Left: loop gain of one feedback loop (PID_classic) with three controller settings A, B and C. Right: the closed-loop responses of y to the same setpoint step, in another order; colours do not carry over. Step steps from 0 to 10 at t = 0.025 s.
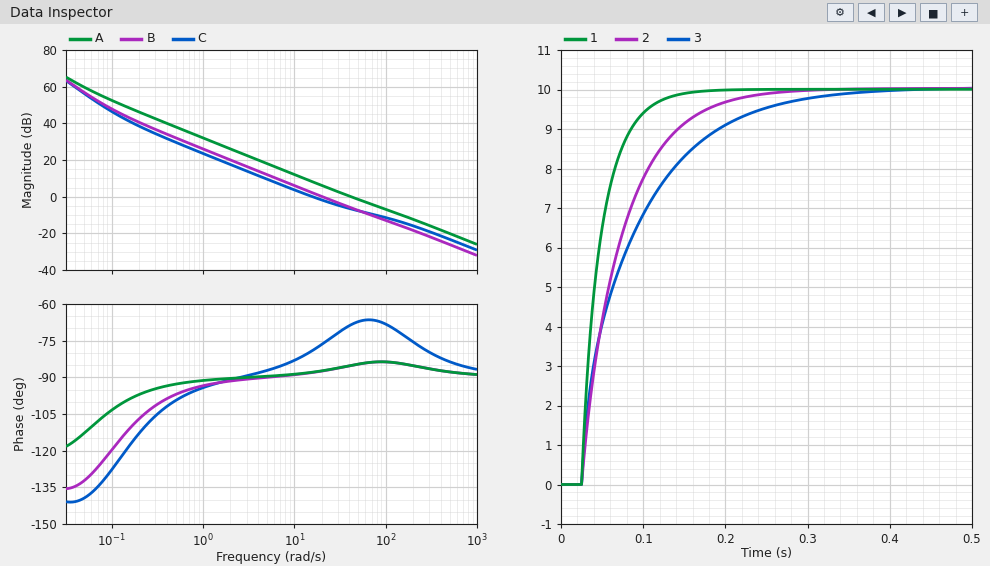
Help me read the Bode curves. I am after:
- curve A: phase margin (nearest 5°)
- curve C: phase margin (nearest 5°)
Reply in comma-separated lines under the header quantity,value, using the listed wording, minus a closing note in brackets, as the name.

quantity,value
curve A: phase margin,95°
curve C: phase margin,100°
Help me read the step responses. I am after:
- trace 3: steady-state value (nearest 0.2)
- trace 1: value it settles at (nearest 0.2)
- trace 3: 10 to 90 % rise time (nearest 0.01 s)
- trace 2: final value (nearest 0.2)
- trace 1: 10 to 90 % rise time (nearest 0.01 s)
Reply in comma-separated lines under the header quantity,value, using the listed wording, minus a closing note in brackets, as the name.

quantity,value
trace 3: steady-state value,10.0
trace 1: value it settles at,10.0
trace 3: 10 to 90 % rise time,0.17 s
trace 2: final value,10.0
trace 1: 10 to 90 % rise time,0.06 s
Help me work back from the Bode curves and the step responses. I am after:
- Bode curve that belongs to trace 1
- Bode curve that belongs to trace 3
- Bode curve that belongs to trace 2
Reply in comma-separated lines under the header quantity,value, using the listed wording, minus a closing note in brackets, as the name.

quantity,value
Bode curve that belongs to trace 1,A
Bode curve that belongs to trace 3,C
Bode curve that belongs to trace 2,B
